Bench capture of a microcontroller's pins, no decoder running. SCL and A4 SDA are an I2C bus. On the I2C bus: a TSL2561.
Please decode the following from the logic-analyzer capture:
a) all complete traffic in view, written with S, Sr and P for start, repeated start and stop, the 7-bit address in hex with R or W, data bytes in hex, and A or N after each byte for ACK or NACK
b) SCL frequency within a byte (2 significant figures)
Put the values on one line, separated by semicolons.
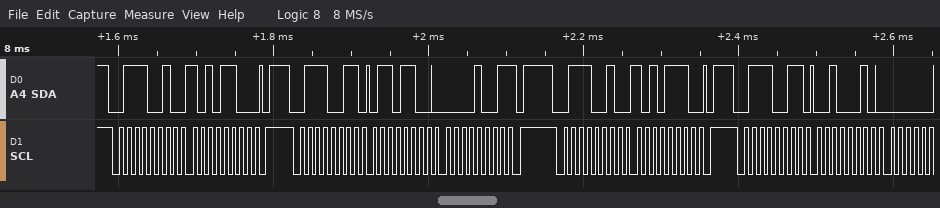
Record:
S 39W A AC A P S 39R A 6C A 09 N P S 39W A AE A P S 39R A 22 A; 100 kHz
